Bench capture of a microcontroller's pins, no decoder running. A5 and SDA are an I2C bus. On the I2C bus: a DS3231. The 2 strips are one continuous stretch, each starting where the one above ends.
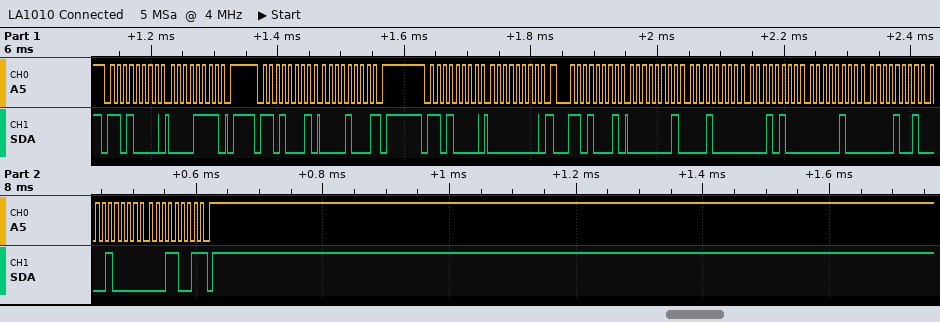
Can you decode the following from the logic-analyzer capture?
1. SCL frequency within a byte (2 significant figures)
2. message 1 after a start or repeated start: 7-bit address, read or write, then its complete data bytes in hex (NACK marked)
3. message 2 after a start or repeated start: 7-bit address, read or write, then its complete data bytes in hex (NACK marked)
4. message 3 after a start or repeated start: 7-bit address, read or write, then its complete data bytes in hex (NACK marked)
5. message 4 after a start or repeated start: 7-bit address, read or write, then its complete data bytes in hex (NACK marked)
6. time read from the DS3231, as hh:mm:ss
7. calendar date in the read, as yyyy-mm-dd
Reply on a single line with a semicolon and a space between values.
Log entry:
100 kHz; 0x68 write: 0F; 0x68 read: 08 NACK; 0x68 write: 00; 0x68 read: 01 10 14 04 09 10 19 NACK; 14:10:01; 2019-10-09
